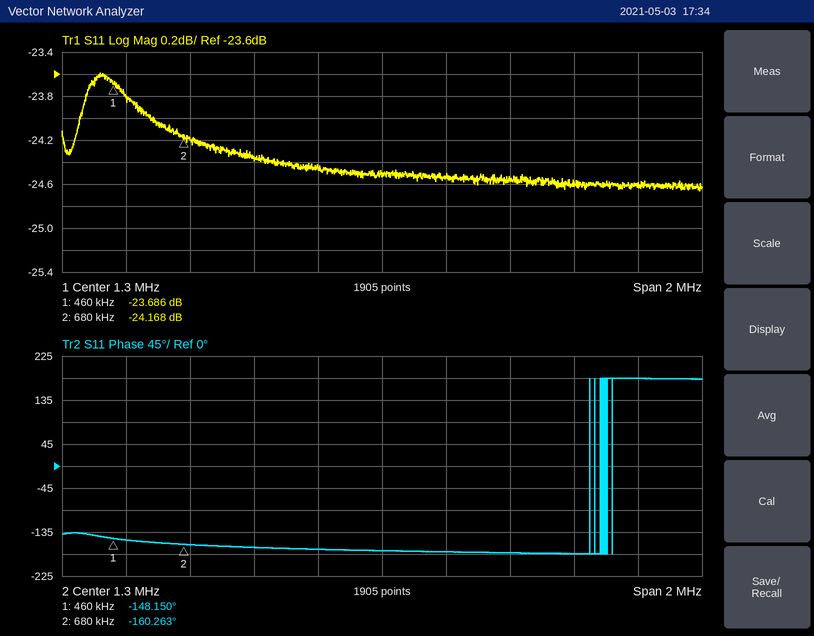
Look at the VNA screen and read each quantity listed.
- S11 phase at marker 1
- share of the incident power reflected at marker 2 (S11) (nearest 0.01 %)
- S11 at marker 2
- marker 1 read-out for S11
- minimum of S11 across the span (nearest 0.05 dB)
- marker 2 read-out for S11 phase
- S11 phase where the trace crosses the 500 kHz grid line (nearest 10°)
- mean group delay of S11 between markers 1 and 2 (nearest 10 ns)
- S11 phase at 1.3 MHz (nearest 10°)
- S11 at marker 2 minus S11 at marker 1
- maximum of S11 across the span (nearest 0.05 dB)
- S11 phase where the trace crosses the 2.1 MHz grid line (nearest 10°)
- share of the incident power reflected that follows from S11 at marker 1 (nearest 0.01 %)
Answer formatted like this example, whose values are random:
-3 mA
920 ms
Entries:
-148.150°
0.38 %
-24.168 dB
-23.686 dB
-24.65 dB
-160.263°
-150°
150 ns
-170°
-0.482 dB
-23.60 dB
180°
0.43 %
